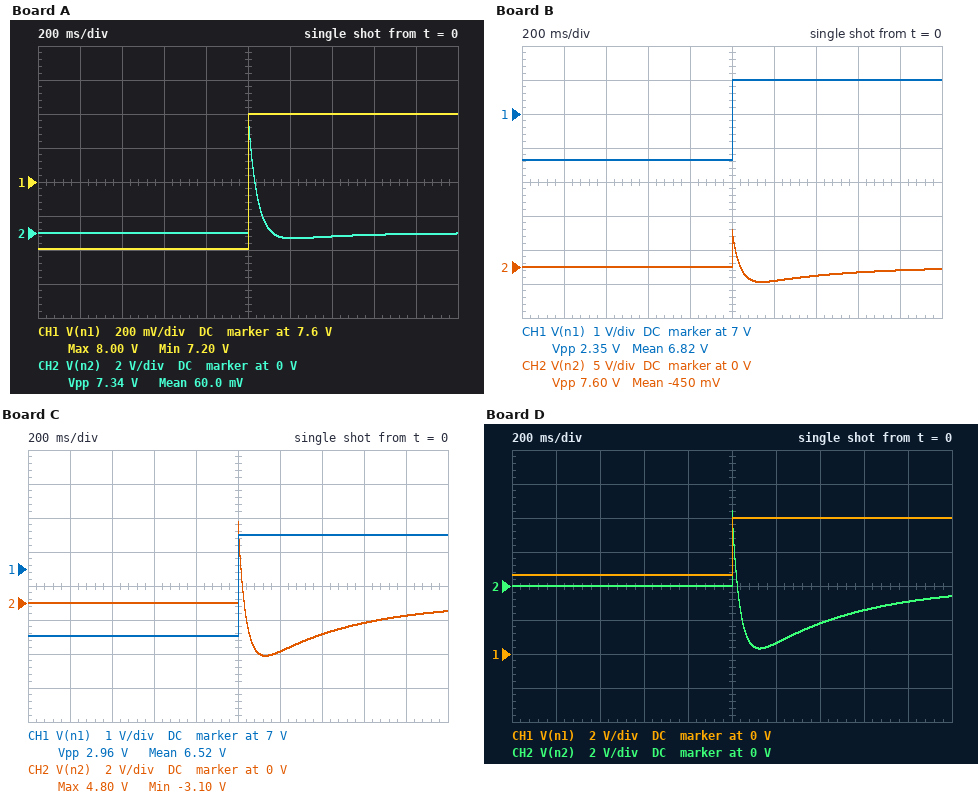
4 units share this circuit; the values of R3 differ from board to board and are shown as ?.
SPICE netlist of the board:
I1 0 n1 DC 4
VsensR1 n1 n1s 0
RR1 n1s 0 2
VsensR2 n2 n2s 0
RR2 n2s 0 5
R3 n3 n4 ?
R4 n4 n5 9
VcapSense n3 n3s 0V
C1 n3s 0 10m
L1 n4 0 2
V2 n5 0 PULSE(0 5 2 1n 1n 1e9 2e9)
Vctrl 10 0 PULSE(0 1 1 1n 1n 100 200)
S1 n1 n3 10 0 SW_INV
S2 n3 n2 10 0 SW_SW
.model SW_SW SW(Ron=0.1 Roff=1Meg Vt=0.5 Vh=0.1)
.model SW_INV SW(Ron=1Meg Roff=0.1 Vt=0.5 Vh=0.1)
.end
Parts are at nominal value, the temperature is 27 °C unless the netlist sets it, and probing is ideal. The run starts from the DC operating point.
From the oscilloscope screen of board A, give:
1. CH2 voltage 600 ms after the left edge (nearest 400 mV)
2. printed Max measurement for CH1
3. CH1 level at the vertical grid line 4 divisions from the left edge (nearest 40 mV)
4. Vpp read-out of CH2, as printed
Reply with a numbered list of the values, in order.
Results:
1. 0 V
2. 8.00 V
3. 7.20 V
4. 7.34 V
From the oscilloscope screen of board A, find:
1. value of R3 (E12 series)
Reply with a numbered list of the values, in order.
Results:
1. 18 Ω
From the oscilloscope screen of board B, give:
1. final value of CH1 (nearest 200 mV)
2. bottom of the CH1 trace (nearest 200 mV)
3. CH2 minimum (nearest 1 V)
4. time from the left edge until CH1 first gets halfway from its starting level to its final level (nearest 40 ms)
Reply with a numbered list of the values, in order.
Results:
1. 8.0 V
2. 5.6 V
3. -2 V
4. 1.00 s
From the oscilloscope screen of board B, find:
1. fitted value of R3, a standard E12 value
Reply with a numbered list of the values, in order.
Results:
1. 4.7 Ω
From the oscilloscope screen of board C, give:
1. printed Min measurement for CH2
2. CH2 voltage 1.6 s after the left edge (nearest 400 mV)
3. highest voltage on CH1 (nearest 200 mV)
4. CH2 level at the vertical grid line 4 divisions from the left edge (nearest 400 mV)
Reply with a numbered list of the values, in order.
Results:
1. -3.10 V
2. -1.2 V
3. 8.0 V
4. 0 V
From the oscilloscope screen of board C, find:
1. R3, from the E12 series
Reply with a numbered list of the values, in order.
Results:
1. 3.3 Ω
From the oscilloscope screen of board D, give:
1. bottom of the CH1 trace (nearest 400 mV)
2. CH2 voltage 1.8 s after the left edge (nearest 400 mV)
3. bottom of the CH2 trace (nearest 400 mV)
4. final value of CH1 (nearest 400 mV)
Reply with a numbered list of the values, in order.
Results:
1. 4.8 V
2. -800 mV
3. -3.6 V
4. 8.0 V
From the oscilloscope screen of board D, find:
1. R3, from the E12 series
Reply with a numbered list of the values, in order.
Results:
1. 2.7 Ω
